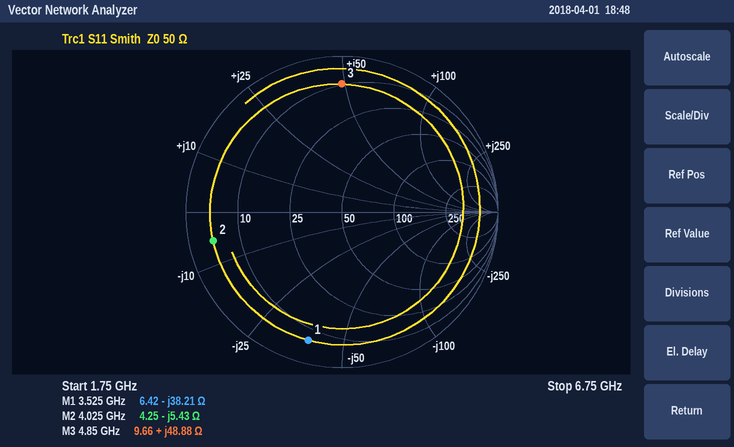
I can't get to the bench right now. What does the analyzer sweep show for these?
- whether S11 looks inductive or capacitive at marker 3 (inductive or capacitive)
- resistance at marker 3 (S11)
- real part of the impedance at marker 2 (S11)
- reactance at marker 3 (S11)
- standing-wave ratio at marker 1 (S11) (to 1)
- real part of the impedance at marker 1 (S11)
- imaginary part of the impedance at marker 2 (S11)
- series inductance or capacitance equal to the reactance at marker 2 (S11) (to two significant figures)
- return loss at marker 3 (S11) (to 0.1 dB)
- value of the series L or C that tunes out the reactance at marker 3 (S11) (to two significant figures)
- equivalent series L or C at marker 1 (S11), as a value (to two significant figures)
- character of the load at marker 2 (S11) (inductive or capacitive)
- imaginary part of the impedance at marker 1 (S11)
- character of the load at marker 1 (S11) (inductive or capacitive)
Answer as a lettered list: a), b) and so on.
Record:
a) inductive
b) 9.66 Ω
c) 4.25 Ω
d) +48.88 Ω
e) 12
f) 6.42 Ω
g) -5.43 Ω
h) 7.3 pF
i) 1.7 dB
j) 670 fF
k) 1.2 pF
l) capacitive
m) -38.21 Ω
n) capacitive
